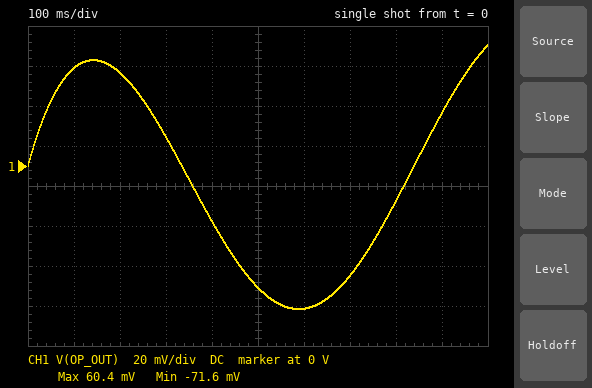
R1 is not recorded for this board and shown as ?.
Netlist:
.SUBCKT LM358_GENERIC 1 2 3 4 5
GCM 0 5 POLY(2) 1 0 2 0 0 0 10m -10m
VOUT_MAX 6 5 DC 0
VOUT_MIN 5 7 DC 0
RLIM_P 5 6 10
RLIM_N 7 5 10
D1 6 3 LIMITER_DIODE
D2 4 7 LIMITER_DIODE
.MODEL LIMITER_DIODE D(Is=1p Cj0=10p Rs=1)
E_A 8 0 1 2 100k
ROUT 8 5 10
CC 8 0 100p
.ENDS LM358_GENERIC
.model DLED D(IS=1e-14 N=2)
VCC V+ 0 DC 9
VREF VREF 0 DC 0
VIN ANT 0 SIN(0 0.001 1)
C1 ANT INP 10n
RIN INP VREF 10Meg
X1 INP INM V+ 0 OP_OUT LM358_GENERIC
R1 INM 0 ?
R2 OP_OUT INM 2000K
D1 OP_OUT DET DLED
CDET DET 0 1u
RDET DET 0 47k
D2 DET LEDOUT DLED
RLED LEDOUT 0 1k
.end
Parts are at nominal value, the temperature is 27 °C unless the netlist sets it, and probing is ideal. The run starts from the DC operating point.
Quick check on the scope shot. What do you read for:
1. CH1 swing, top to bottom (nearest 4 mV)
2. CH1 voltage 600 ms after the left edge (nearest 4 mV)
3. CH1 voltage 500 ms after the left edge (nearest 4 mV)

132 mV
-72 mV
-60 mV
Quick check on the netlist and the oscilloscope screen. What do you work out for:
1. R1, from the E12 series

15 kΩ
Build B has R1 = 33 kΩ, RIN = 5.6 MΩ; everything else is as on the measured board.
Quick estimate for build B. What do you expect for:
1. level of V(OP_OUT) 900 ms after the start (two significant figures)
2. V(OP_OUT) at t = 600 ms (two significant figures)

12 mV
-20 mV
